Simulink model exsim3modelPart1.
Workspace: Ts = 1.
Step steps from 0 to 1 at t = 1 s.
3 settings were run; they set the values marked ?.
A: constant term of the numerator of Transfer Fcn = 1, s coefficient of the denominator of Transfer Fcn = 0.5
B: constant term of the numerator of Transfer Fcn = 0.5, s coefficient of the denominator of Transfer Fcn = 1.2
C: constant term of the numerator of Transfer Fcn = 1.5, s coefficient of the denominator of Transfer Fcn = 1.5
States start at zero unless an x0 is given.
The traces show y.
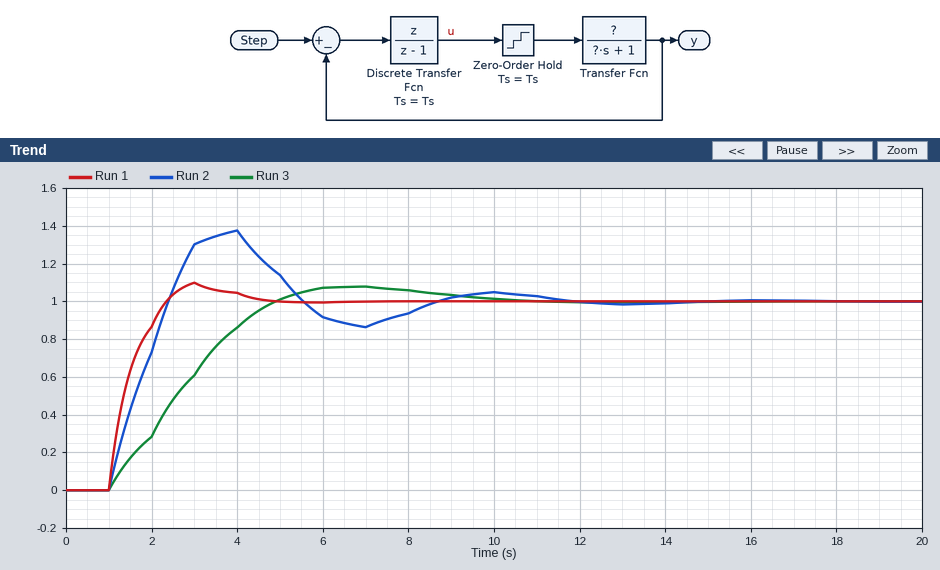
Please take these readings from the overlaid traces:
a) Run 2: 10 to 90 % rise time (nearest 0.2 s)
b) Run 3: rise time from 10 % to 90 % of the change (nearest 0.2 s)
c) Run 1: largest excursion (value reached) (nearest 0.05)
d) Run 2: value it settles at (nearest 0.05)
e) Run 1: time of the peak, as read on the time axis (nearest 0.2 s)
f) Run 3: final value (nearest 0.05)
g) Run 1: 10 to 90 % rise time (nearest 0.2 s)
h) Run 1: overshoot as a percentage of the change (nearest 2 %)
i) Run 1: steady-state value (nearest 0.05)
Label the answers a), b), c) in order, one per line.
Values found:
a) 1.2 s
b) 3.0 s
c) 1.10
d) 1.00
e) 3.0 s
f) 1.00
g) 1.0 s
h) 10 %
i) 1.00
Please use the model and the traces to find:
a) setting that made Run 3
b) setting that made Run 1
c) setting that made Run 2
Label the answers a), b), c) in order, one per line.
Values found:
a) B
b) A
c) C
